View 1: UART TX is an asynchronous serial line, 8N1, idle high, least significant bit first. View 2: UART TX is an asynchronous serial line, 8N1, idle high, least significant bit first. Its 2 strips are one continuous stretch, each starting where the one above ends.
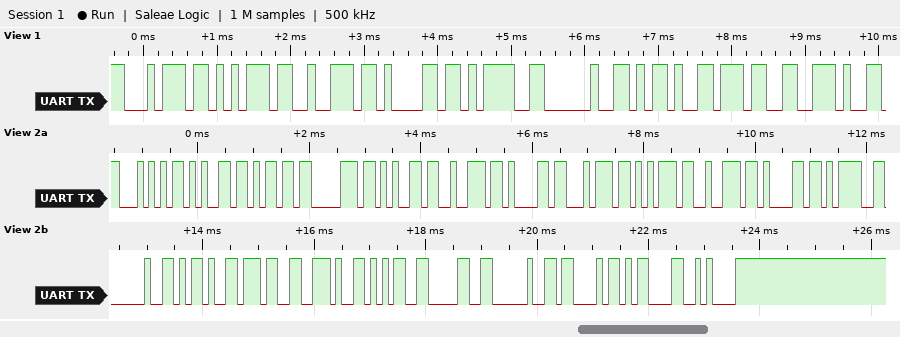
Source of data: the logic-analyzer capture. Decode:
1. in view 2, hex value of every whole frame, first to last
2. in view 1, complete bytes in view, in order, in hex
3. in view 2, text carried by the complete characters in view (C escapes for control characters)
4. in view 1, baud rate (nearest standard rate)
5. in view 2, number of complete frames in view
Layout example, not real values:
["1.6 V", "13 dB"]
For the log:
["54 65 6D 70 65 72 61 74 75 72 61 3D 20 2D 37 2E 35 30 20 43 0D 0A", "74 75 72 61 3D 20 2D 37 2E", "\"Temperatura= -7.50 C\\r\\n\"", "9600 baud", "22"]
